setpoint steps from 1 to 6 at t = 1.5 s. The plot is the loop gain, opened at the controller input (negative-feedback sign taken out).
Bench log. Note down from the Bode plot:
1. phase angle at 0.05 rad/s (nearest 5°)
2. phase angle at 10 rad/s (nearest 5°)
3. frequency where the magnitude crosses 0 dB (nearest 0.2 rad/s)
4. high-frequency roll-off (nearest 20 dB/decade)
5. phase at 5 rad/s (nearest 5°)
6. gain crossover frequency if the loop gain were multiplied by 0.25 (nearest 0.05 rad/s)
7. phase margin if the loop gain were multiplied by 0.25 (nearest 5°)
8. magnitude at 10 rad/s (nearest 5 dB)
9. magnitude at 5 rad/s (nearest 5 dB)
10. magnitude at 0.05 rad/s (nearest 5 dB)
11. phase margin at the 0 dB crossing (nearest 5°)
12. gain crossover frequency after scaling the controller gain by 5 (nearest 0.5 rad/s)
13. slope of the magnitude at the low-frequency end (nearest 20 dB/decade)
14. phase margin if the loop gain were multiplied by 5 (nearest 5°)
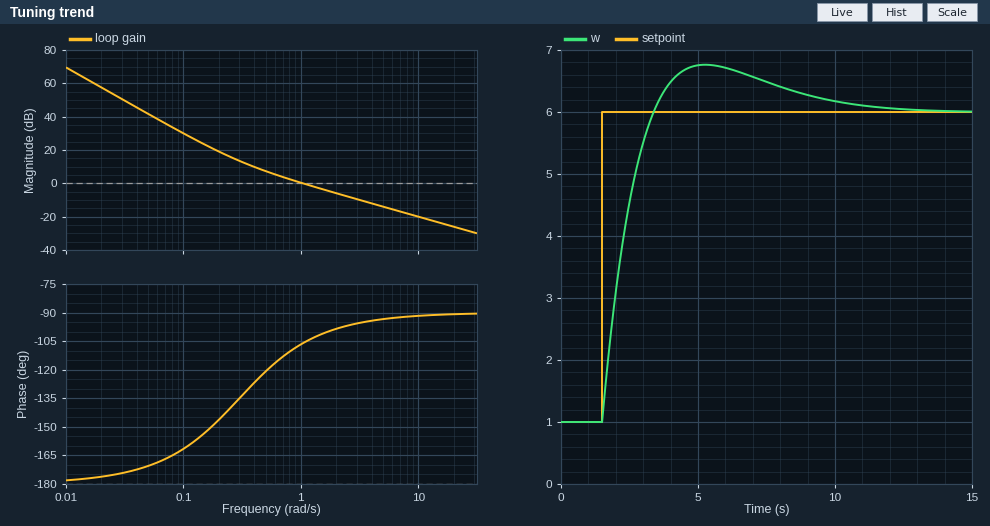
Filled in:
-170°
-90°
1.0 rad/s
-20 dB/decade
-95°
0.35 rad/s
50°
-20 dB
-15 dB
40 dB
75°
5.0 rad/s
-40 dB/decade
85°
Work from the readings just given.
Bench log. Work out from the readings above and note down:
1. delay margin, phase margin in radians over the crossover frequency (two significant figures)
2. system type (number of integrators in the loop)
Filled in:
1.3 s
2
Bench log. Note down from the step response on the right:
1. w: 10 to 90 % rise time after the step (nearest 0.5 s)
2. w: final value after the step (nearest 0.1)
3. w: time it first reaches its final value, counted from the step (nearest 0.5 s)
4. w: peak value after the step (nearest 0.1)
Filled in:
1.5 s
6.0
2.0 s
6.8
